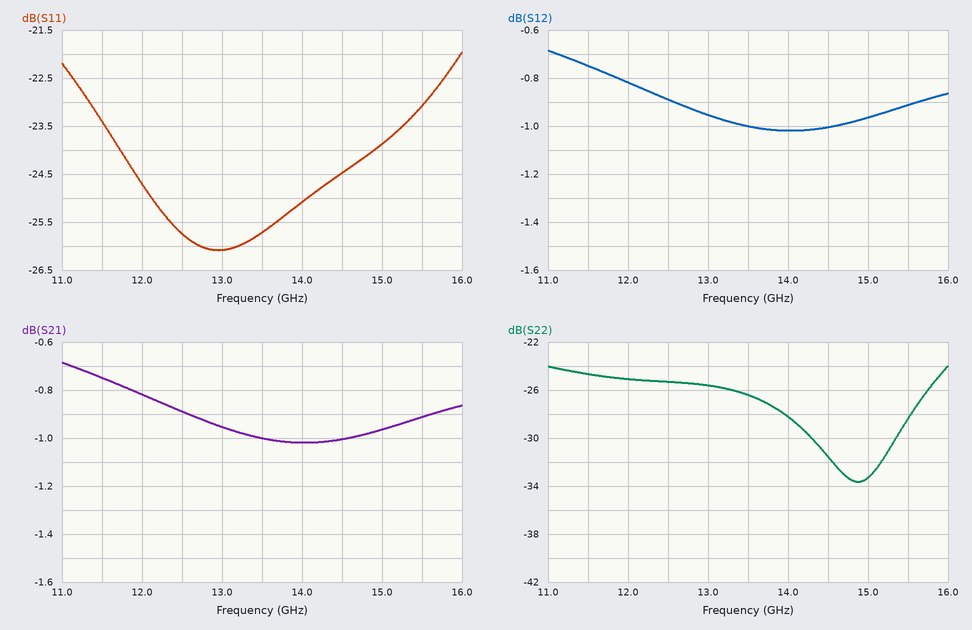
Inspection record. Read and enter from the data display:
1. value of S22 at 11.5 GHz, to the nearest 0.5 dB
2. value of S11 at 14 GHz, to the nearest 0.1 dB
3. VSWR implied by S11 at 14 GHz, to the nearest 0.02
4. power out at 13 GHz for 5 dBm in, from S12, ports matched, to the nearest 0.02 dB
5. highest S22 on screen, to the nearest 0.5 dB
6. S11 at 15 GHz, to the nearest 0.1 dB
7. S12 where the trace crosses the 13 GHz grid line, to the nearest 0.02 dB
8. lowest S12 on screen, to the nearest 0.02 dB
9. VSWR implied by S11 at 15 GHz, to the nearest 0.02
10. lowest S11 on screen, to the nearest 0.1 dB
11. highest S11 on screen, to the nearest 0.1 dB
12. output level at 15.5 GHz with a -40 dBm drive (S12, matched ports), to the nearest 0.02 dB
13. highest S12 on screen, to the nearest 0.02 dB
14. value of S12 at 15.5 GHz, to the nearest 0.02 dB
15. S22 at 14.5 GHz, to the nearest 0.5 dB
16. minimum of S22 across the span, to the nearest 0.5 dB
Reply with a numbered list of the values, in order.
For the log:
1. -24.5 dB
2. -25.1 dB
3. 1.12
4. 4.04 dBm
5. -24.0 dB
6. -23.9 dB
7. -0.96 dB
8. -1.02 dB
9. 1.14
10. -26.1 dB
11. -22.0 dB
12. -40.92 dBm
13. -0.68 dB
14. -0.92 dB
15. -31.5 dB
16. -33.5 dB
